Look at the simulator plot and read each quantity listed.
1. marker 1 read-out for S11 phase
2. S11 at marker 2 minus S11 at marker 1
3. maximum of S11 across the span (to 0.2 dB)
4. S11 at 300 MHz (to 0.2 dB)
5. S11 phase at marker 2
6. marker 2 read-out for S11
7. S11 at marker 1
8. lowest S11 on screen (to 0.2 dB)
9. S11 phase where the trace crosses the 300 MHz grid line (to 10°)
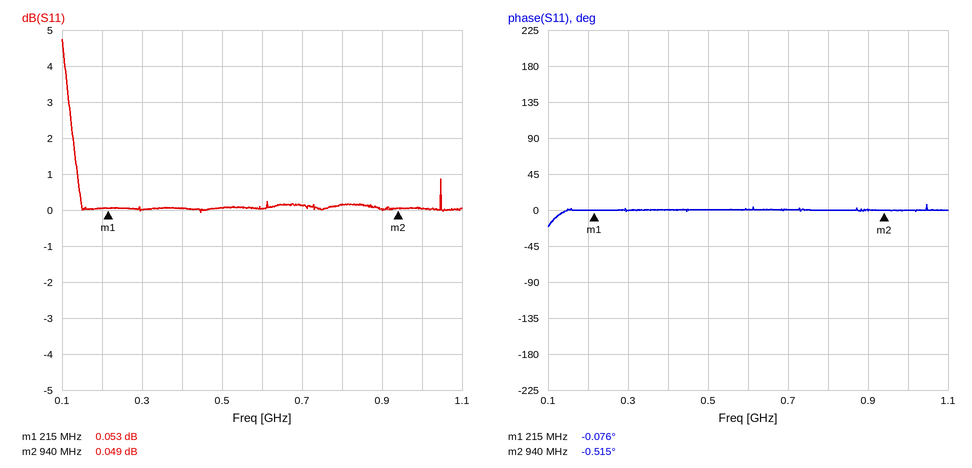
-0.076°
-0.004 dB
4.8 dB
0.0 dB
-0.515°
0.049 dB
0.053 dB
0.0 dB
0°
